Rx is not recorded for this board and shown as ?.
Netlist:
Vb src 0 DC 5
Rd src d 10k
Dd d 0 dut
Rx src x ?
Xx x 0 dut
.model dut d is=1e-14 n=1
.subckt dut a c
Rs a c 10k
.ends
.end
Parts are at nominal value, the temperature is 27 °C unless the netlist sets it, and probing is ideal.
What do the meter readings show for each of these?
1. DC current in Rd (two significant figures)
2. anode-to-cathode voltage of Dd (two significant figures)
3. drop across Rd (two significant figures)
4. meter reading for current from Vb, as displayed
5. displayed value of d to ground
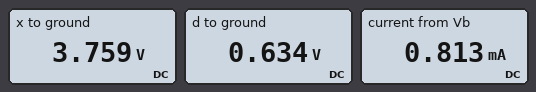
440 µA
630 mV
4.4 V
0.813 mA
0.634 V
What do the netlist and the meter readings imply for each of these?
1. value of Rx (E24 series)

3.3 kΩ
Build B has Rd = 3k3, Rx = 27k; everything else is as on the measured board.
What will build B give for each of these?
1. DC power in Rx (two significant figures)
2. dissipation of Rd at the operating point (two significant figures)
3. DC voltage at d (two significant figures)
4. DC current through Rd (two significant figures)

490 µW
5.7 mW
660 mV
1.3 mA
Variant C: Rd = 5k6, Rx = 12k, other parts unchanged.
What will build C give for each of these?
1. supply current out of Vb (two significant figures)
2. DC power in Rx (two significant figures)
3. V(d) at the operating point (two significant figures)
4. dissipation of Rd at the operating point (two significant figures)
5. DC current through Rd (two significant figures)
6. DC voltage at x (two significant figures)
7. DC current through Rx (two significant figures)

1.0 mA
620 µW
650 mV
3.4 mW
780 µA
2.3 V
230 µA
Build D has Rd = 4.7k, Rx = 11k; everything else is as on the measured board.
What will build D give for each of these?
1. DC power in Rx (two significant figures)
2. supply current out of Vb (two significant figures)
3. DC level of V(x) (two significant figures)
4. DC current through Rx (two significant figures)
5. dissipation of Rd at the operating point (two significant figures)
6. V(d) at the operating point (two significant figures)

620 µW
1.2 mA
2.4 V
240 µA
4.0 mW
650 mV
